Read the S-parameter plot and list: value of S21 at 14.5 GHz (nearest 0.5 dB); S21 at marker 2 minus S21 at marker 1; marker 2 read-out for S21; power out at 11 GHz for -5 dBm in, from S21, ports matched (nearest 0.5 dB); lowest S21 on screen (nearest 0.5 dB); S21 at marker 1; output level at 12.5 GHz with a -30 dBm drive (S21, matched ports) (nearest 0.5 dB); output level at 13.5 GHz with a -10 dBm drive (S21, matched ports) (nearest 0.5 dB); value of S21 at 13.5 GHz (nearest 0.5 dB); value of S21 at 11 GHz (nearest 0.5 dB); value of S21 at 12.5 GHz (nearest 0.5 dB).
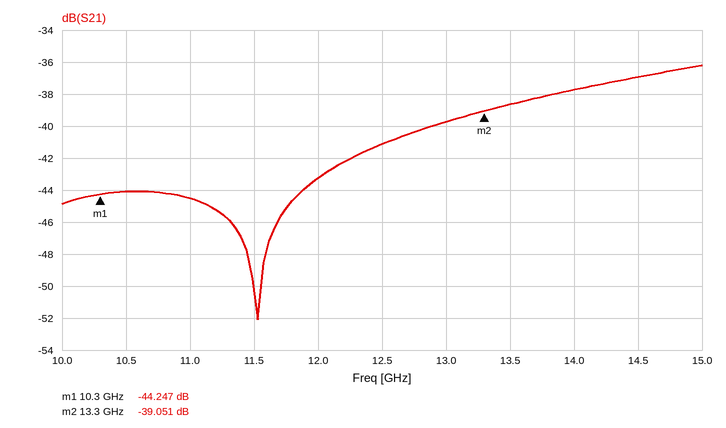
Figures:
-37.0 dB
5.196 dB
-39.051 dB
-49.5 dBm
-52.0 dB
-44.247 dB
-71.0 dBm
-48.5 dBm
-38.5 dB
-44.5 dB
-41.0 dB
